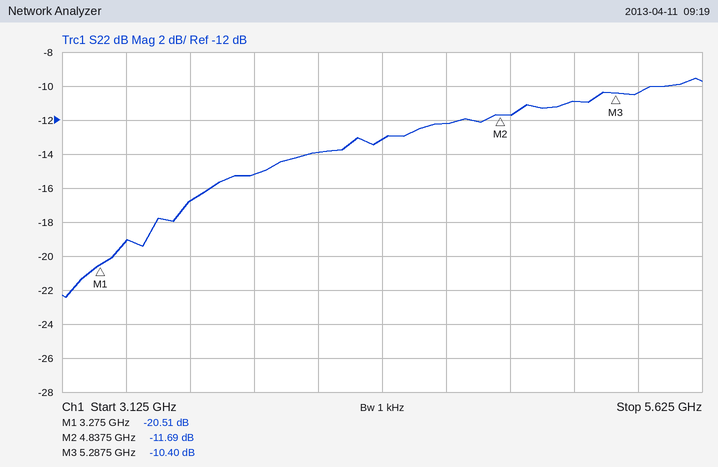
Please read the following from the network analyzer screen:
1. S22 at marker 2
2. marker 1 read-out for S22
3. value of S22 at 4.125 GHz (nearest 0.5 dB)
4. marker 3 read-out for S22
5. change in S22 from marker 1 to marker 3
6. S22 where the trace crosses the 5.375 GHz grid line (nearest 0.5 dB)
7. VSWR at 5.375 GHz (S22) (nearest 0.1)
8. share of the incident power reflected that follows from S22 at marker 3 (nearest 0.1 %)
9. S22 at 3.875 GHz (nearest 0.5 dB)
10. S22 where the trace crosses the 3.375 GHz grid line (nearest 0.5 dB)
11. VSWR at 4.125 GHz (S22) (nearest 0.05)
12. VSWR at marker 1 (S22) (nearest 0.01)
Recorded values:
-11.69 dB
-20.51 dB
-14.0 dB
-10.40 dB
10.11 dB
-10.5 dB
1.9
9.1 %
-15.0 dB
-19.0 dB
1.50
1.21
